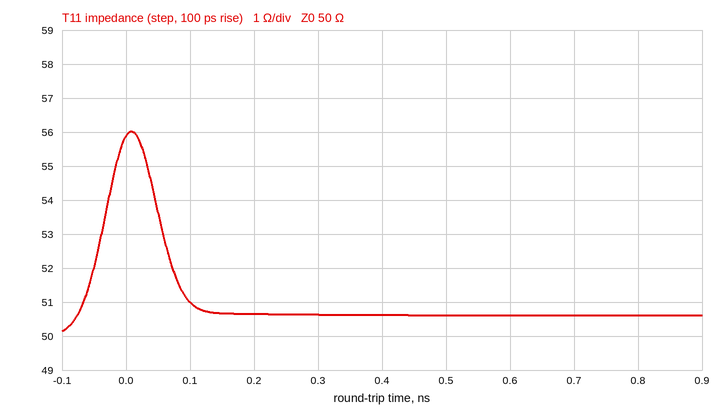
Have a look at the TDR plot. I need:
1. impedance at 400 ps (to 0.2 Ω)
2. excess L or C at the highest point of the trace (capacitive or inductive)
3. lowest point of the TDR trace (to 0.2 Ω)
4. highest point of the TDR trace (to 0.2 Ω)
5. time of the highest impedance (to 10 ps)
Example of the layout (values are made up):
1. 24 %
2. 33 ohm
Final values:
1. 50.6 Ω
2. inductive
3. 50.2 Ω
4. 56.0 Ω
5. 10 ps
